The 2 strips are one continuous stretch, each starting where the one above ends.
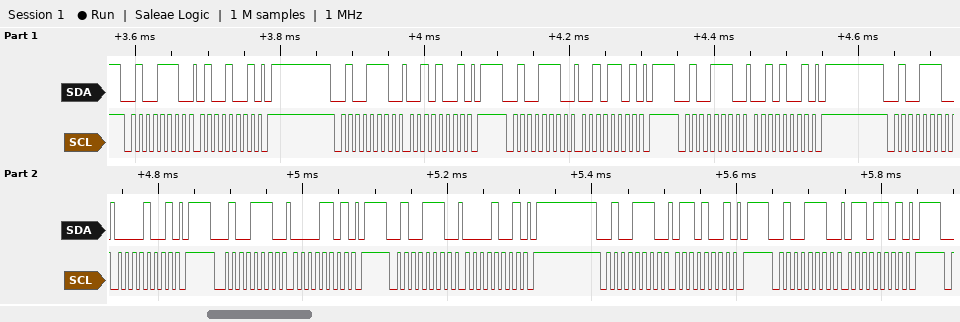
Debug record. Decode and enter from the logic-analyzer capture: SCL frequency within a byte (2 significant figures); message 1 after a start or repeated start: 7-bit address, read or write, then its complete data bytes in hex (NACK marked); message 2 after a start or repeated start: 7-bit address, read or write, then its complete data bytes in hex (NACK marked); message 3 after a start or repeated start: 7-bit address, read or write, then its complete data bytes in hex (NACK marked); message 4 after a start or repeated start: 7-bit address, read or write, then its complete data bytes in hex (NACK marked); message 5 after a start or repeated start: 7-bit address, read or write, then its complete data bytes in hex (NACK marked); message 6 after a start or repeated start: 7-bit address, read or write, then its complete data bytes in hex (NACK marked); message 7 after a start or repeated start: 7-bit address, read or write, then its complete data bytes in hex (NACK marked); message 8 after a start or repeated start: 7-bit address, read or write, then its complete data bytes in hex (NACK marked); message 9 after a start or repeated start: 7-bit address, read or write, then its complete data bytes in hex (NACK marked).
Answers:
100 kHz
0x27 write: 49
0x27 write: 29
0x27 write: 2D
0x27 write: 29
0x27 write: 09
0x27 write: 0D
0x27 write: 09
0x27 write: 69
0x27 write: 6D
